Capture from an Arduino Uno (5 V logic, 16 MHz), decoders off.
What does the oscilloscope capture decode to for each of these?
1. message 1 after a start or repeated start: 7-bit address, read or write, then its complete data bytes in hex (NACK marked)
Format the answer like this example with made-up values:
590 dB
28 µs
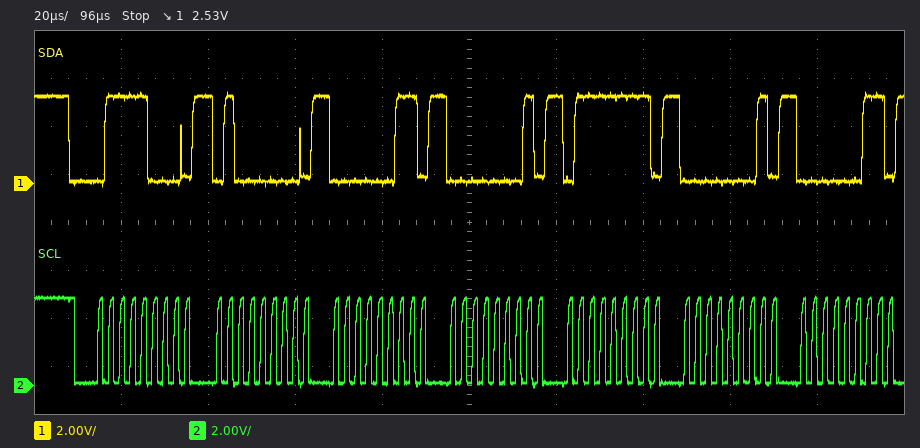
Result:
0x3C write: 40 03 01 7F 01 03
